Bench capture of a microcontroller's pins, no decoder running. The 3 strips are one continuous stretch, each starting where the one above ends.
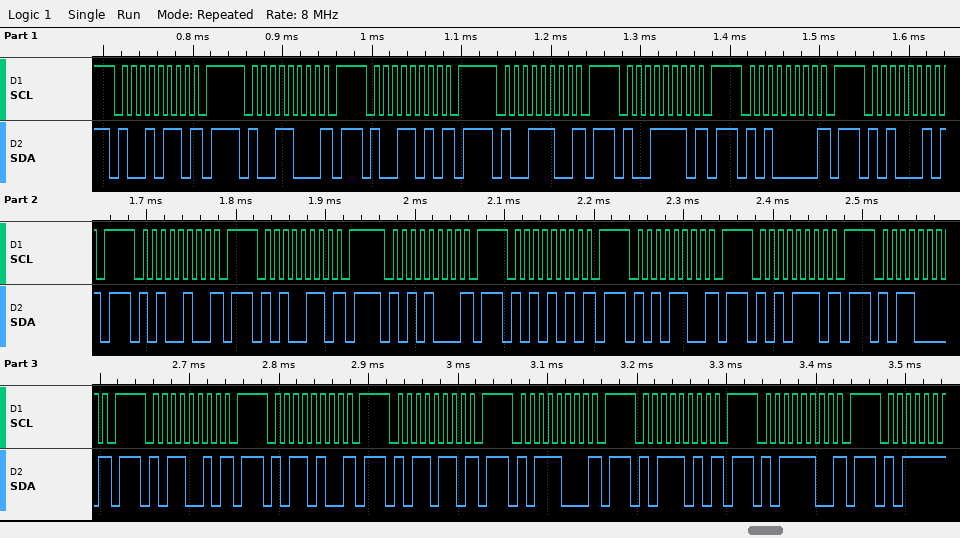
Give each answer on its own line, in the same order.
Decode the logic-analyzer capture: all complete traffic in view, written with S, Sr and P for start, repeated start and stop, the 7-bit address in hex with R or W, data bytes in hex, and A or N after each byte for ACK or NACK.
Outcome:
S 4BW N P S 4CW N P S 4DW N P S 4EW N P S 4FW N P S 50W N P S 51W N P S 52W N P S 53W N P S 54W N P S 55W N P S 56W N P S 57W N P S 58W N P S 59W N P S 5AW N P S 5BW N P S 5CW N P S 5DW N P S 5EW N P
